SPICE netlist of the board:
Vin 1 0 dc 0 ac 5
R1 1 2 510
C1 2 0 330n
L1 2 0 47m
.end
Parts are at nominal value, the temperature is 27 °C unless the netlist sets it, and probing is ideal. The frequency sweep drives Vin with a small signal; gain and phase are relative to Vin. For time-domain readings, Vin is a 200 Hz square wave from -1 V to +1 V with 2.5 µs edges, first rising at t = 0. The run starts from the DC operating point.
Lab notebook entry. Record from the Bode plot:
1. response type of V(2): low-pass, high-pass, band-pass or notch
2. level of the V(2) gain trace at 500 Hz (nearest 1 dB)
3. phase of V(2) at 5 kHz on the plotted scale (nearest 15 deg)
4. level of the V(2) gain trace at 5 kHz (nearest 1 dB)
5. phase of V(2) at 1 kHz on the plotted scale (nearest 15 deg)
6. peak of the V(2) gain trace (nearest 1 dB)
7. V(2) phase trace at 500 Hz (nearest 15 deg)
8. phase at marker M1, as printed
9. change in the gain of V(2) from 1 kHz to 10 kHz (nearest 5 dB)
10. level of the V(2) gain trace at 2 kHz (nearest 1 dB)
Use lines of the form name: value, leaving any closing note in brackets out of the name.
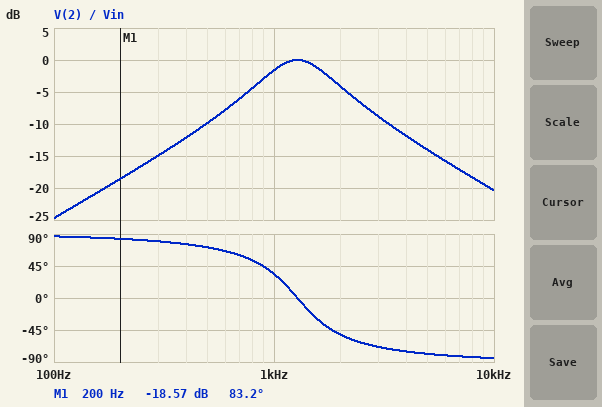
response type of V(2): low-pass, high-pass, band-pass or notch: band-pass
level of the V(2) gain trace at 500 Hz: -10 dB
phase of V(2) at 5 kHz on the plotted scale: -75 deg
level of the V(2) gain trace at 5 kHz: -14 dB
phase of V(2) at 1 kHz on the plotted scale: 30 deg
peak of the V(2) gain trace: 0 dB
V(2) phase trace at 500 Hz: 75 deg
phase at marker M1, as printed: 83.2 deg
change in the gain of V(2) from 1 kHz to 10 kHz: -20 dB
level of the V(2) gain trace at 2 kHz: -4 dB
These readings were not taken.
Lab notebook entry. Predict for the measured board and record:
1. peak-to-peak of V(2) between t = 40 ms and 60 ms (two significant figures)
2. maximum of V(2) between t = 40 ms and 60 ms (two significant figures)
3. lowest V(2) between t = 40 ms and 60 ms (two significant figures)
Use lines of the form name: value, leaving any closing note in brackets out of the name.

peak-to-peak of V(2) between t = 40 ms and 60 ms: 1.8 V
maximum of V(2) between t = 40 ms and 60 ms: 920 mV
lowest V(2) between t = 40 ms and 60 ms: -920 mV
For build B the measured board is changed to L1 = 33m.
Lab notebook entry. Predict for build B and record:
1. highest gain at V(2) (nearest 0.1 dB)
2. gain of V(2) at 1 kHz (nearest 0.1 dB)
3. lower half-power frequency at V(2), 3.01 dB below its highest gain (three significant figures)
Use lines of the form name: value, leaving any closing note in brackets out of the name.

highest gain at V(2): 0 dB
gain of V(2) at 1 kHz: -4.7 dB
lower half-power frequency at V(2), 3.01 dB below its highest gain: 1.12 kHz
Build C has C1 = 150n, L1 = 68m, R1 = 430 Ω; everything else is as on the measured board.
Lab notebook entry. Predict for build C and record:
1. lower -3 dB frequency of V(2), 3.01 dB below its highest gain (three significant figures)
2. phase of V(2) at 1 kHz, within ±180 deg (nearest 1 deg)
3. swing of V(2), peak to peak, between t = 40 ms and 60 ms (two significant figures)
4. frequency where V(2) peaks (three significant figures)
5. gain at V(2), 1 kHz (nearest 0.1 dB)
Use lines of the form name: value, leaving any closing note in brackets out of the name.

lower -3 dB frequency of V(2), 3.01 dB below its highest gain: 768 Hz
phase of V(2) at 1 kHz, within ±180 deg: 31 deg
swing of V(2), peak to peak, between t = 40 ms and 60 ms: 2.7 V
frequency where V(2) peaks: 1.58 kHz
gain at V(2), 1 kHz: -1.3 dB
